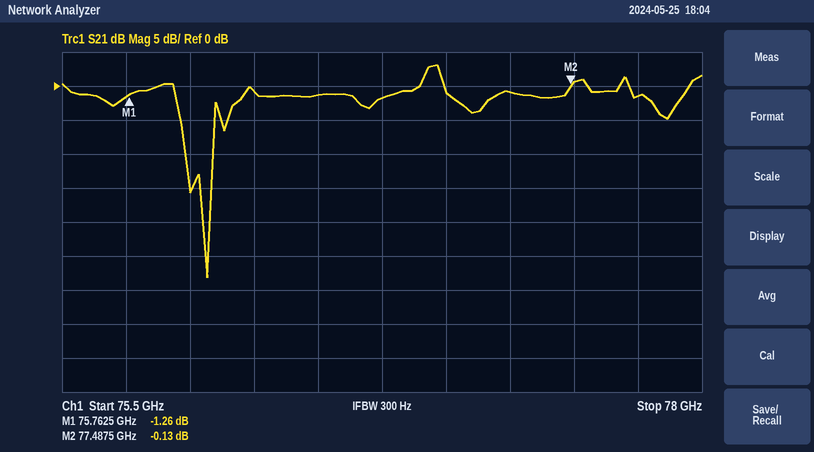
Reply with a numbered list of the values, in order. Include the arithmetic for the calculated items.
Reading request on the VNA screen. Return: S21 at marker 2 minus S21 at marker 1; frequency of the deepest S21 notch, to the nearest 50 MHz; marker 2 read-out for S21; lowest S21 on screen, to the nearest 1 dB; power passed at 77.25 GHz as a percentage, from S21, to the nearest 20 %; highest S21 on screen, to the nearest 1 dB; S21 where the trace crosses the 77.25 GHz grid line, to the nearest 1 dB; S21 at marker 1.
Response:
1. -0.13 − (-1.26) = 1.13 dB
2. 76.05 GHz
3. -0.13 dB
4. -28 dB
5. 10^(-1/10) ≈ 79.4 %, so 80 % to the nearest 20 %
6. 3 dB
7. -1 dB
8. -1.26 dB
